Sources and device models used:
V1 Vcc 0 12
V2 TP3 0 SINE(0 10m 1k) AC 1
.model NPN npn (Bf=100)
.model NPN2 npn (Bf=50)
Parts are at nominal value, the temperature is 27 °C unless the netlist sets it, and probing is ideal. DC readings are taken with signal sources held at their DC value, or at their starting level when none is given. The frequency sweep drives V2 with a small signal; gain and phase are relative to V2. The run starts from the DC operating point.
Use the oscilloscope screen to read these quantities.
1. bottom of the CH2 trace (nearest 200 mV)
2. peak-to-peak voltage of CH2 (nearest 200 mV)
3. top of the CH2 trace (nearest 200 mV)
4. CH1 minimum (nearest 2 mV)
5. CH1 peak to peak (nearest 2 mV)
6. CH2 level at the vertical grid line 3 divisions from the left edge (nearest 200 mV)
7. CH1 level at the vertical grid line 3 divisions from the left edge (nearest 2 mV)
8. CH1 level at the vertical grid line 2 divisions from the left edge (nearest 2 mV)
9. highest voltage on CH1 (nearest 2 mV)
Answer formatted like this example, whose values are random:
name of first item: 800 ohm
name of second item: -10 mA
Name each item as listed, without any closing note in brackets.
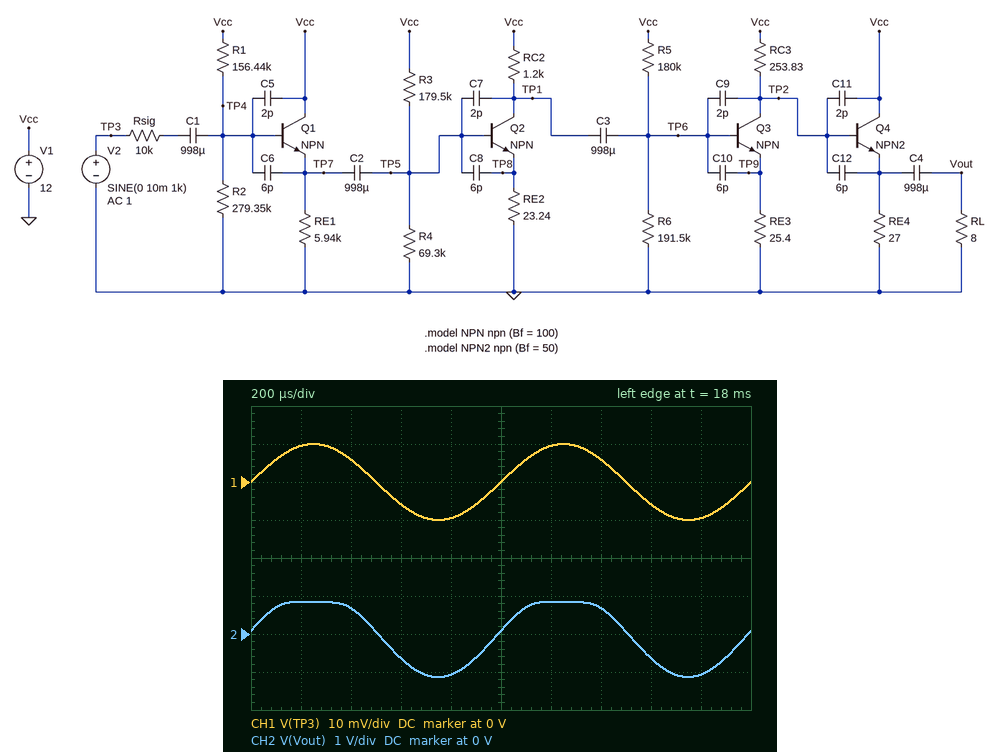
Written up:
bottom of the CH2 trace: -1.2 V
peak-to-peak voltage of CH2: 2.0 V
top of the CH2 trace: 800 mV
CH1 minimum: -10 mV
CH1 peak to peak: 20 mV
CH2 level at the vertical grid line 3 divisions from the left edge: -600 mV
CH1 level at the vertical grid line 3 divisions from the left edge: -6 mV
CH1 level at the vertical grid line 2 divisions from the left edge: 6 mV
highest voltage on CH1: 10 mV
